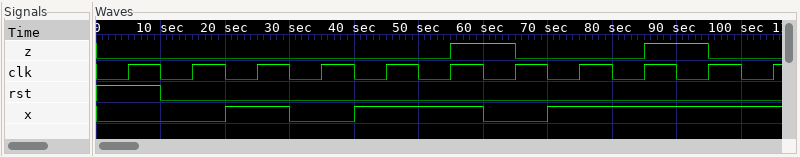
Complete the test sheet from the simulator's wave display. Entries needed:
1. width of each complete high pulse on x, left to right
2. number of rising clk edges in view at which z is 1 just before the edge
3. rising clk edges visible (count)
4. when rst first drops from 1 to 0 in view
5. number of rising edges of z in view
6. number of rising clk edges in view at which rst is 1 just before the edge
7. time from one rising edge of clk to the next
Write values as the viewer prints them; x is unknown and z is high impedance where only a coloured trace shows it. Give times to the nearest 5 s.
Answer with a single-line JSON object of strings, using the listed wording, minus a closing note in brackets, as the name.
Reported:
{"width of each complete high pulse on x, left to right": "10 s, 20 s", "number of rising clk edges in view at which z is 1 just before the edge": "2", "rising clk edges visible": "11", "when rst first drops from 1 to 0 in view": "10 s", "number of rising edges of z in view": "2", "number of rising clk edges in view at which rst is 1 just before the edge": "1", "time from one rising edge of clk to the next": "10 s"}
